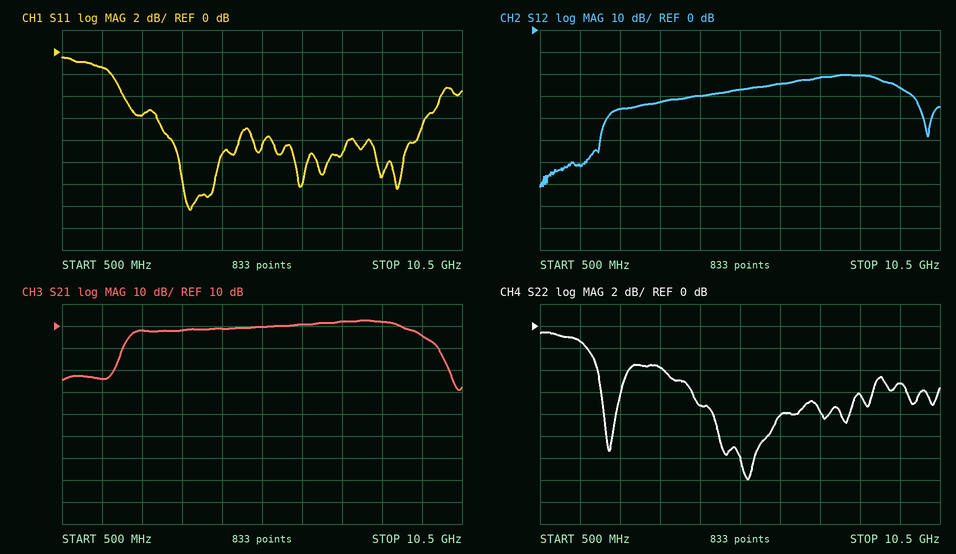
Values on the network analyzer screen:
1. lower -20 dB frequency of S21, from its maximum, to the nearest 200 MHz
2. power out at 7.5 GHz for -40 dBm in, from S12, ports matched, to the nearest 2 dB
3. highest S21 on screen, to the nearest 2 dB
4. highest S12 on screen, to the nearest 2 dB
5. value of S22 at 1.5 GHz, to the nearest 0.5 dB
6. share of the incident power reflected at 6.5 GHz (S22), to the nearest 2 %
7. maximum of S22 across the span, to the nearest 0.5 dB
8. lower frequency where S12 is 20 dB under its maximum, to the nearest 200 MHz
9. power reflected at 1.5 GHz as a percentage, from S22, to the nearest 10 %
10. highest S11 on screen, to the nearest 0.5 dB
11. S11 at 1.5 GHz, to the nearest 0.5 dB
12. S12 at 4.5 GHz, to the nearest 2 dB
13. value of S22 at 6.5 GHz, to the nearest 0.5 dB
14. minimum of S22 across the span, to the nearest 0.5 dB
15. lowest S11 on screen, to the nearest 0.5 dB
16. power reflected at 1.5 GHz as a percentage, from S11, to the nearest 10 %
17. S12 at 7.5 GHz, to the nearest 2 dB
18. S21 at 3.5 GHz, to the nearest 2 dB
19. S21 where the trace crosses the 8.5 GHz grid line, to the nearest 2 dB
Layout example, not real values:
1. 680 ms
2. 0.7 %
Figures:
1. 1.8 GHz
2. -62 dBm
3. 12 dB
4. -20 dB
5. -1.5 dB
6. 16 %
7. -0.5 dB
8. 2.2 GHz
9. 70 %
10. -0.5 dB
11. -1.5 dB
12. -30 dB
13. -8.0 dB
14. -14.0 dB
15. -14.5 dB
16. 70 %
17. -22 dB
18. 8 dB
19. 12 dB
